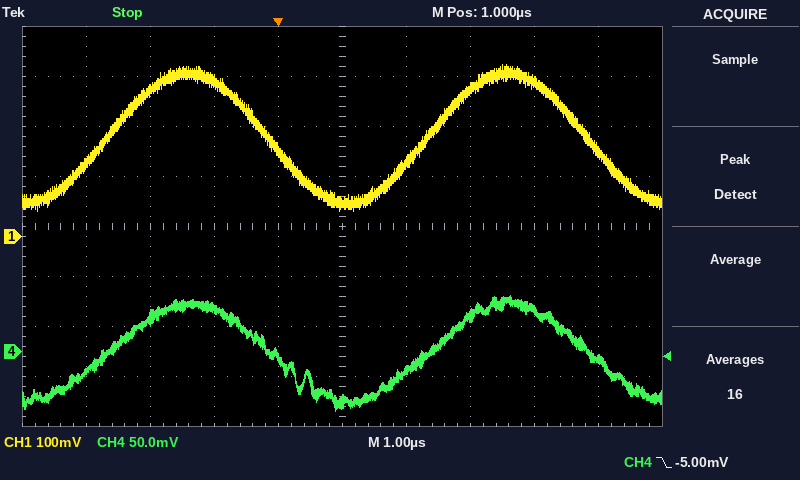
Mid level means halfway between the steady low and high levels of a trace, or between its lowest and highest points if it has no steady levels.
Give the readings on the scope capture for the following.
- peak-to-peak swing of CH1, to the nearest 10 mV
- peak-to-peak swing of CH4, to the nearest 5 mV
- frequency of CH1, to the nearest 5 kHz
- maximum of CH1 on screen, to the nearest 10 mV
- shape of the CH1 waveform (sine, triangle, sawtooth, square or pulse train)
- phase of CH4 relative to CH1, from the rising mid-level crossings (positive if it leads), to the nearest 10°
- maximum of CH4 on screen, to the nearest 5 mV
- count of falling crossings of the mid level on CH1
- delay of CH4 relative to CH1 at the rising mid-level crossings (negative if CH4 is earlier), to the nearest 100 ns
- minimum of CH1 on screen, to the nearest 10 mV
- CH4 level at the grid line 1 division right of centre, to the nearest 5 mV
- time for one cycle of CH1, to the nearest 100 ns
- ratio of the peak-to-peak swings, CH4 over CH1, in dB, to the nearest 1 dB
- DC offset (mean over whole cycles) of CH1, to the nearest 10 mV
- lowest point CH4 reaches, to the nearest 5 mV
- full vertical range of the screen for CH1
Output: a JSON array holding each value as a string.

["290 mV", "115 mV", "200 kHz", "340 mV", "sine", "0°", "55 mV", "2", "0.0 µs", "50 mV", "-20 mV", "5.0 µs", "-8 dB", "200 mV", "-60 mV", "800 mV"]
